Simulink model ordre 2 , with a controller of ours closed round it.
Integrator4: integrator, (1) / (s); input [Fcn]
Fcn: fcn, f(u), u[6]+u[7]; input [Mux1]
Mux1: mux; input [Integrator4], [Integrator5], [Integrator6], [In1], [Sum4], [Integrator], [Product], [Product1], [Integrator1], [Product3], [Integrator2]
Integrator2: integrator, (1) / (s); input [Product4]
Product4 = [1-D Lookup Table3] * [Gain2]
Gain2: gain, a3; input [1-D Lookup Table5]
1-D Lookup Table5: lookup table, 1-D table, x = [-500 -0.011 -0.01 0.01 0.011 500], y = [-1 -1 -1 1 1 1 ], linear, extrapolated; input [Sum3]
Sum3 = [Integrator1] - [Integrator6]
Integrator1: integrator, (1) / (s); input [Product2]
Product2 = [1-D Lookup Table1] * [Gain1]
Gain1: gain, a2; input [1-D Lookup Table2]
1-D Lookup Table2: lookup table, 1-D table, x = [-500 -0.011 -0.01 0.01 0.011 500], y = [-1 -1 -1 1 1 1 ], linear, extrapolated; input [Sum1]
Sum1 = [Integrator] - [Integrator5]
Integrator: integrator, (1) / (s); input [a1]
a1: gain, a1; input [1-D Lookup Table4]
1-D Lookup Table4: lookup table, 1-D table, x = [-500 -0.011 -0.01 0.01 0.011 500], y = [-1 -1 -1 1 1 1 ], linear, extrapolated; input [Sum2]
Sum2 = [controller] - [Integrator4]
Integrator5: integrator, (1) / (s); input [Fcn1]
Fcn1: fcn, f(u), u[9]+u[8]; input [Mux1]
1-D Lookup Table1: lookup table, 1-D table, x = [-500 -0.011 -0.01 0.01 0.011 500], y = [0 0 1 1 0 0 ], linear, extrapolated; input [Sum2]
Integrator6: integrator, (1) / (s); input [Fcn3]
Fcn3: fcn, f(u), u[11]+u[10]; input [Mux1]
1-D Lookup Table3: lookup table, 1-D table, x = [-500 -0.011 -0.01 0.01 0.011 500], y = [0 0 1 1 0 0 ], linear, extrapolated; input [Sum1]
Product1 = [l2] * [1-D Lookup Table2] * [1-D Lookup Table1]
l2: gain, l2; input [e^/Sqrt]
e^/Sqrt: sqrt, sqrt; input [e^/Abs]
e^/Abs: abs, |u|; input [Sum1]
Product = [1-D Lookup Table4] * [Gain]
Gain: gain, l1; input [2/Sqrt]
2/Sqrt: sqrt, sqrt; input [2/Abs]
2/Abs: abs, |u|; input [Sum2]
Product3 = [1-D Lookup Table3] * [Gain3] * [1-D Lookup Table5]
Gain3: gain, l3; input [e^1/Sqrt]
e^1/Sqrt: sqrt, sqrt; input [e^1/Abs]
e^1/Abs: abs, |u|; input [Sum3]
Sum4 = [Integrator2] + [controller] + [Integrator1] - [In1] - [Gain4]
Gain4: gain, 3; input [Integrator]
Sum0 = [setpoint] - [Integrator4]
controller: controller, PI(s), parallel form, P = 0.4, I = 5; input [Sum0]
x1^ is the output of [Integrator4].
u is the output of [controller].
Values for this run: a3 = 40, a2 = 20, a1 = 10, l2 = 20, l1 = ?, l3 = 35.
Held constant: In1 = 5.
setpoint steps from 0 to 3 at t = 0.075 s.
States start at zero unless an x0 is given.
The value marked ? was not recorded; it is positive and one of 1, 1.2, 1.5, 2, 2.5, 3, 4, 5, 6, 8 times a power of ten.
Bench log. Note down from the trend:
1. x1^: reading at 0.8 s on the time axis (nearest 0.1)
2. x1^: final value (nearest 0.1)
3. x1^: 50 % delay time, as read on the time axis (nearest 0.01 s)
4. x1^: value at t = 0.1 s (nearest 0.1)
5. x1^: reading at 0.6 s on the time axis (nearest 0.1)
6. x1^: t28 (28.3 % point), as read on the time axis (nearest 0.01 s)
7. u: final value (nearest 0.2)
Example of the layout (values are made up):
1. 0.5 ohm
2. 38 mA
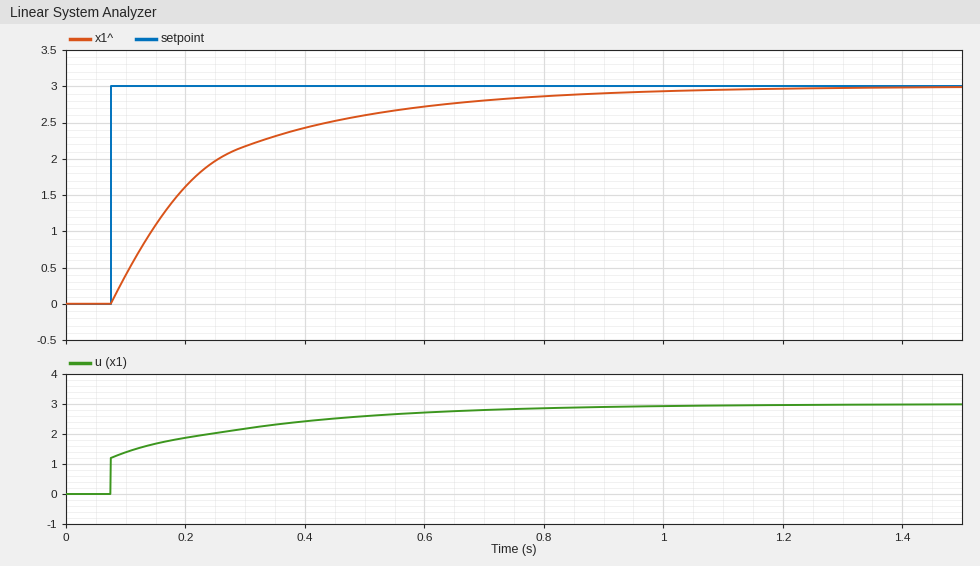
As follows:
1. 2.9
2. 3.0
3. 0.19 s
4. 0.4
5. 2.7
6. 0.13 s
7. 3.0
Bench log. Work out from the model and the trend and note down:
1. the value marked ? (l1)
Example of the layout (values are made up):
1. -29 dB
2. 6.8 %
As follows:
1. 15
